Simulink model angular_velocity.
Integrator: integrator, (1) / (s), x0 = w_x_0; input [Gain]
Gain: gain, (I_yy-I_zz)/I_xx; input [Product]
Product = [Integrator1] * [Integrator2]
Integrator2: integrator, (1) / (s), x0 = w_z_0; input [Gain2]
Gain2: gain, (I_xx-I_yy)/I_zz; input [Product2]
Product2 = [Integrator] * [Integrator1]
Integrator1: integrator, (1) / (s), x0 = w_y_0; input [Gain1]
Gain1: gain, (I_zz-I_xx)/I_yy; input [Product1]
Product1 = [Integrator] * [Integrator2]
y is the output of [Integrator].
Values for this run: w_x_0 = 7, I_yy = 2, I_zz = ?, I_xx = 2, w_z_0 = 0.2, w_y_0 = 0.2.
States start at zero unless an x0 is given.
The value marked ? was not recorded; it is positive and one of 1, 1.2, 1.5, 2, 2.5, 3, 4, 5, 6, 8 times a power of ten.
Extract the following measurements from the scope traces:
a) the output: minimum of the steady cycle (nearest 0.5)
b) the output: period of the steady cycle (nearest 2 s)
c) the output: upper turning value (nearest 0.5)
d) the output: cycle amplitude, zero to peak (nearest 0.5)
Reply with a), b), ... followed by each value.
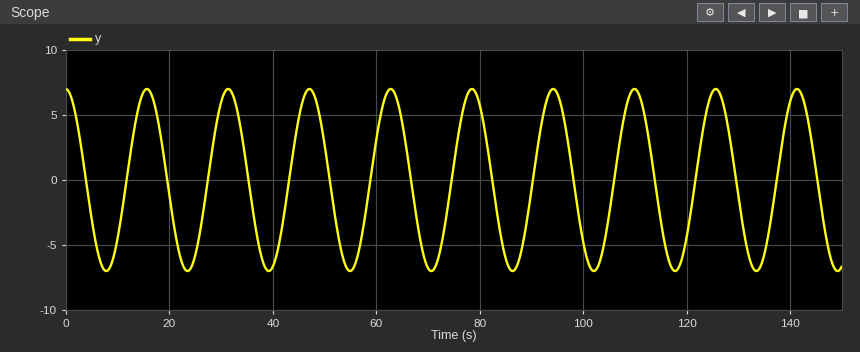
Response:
a) -7.0
b) 16 s
c) 7.0
d) 7.0
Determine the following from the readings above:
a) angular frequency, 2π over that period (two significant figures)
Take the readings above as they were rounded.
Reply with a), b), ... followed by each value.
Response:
a) 0.39 rad/s
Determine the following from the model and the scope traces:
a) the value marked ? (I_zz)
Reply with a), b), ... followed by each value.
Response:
a) 6
